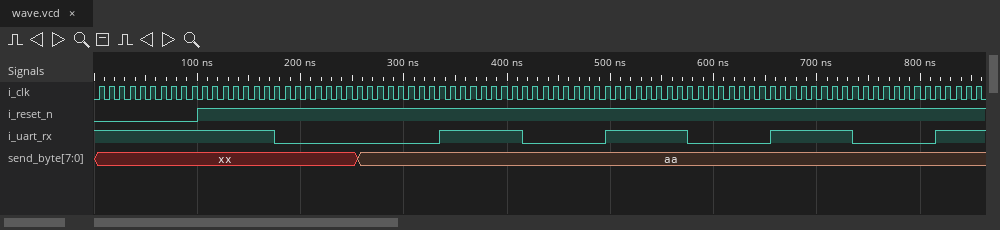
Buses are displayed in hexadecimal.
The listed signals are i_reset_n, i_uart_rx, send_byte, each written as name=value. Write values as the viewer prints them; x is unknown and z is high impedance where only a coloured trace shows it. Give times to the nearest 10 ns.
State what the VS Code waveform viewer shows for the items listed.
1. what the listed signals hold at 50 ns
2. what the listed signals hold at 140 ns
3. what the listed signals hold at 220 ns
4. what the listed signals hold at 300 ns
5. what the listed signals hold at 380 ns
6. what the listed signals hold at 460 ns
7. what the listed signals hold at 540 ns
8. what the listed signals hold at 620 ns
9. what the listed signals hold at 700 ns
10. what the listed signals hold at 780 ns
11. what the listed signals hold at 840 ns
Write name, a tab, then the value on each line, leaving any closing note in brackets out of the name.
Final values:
what the listed signals hold at 50 ns	i_reset_n=0, i_uart_rx=1, send_byte=xx
what the listed signals hold at 140 ns	i_reset_n=1, i_uart_rx=1, send_byte=xx
what the listed signals hold at 220 ns	i_reset_n=1, i_uart_rx=0, send_byte=xx
what the listed signals hold at 300 ns	i_reset_n=1, i_uart_rx=0, send_byte=aa
what the listed signals hold at 380 ns	i_reset_n=1, i_uart_rx=1, send_byte=aa
what the listed signals hold at 460 ns	i_reset_n=1, i_uart_rx=0, send_byte=aa
what the listed signals hold at 540 ns	i_reset_n=1, i_uart_rx=1, send_byte=aa
what the listed signals hold at 620 ns	i_reset_n=1, i_uart_rx=0, send_byte=aa
what the listed signals hold at 700 ns	i_reset_n=1, i_uart_rx=1, send_byte=aa
what the listed signals hold at 780 ns	i_reset_n=1, i_uart_rx=0, send_byte=aa
what the listed signals hold at 840 ns	i_reset_n=1, i_uart_rx=1, send_byte=aa
